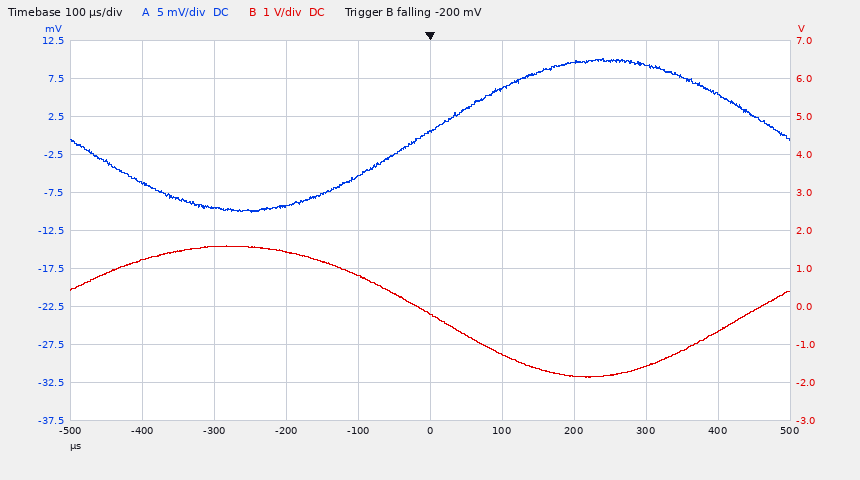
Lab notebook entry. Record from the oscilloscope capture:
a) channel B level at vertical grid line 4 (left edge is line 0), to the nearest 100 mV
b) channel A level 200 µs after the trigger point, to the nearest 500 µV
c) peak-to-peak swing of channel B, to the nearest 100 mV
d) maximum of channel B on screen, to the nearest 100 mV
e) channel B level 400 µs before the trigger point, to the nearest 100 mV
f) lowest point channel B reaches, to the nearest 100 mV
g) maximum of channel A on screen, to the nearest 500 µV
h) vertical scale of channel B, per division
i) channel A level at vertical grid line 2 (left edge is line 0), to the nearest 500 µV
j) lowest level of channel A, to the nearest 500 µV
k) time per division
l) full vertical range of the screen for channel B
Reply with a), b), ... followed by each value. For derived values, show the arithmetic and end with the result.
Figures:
a) 800 mV
b) 9.5 mV
c) 1.6 V − (-1.9 V) = 3.5 V
d) 1.6 V
e) 1.2 V
f) -1.9 V
g) 10.0 mV
h) 1 V
i) -9.5 mV
j) -10.0 mV
k) 100 µs
l) 10 V
